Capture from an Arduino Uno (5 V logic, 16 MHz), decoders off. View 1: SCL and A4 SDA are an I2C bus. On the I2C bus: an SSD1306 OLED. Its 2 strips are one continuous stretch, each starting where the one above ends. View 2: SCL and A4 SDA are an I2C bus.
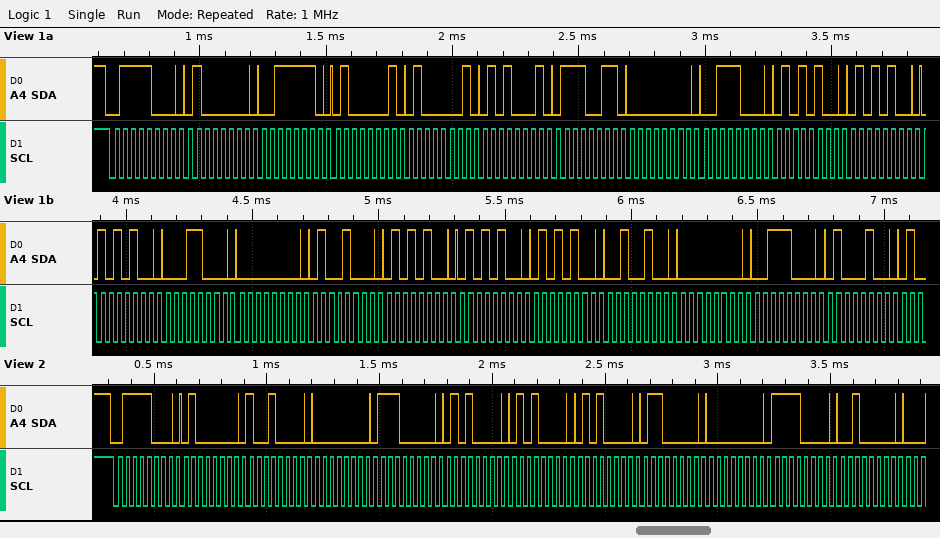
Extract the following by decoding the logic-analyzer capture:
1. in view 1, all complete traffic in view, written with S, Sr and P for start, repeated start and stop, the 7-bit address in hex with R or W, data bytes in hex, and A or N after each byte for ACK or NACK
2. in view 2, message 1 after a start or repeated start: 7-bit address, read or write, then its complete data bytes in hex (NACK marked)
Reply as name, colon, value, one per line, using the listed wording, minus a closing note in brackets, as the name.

in view 1, all complete traffic in view, written with S, Sr and P for start, repeated start and stop, the 7-bit address in hex with R or W, data bytes in hex, and A or N after each byte for ACK or NACK: S 3CW A 40 A 3E A 41 A 41 A 51 A 73 A 00 A 38 A 54 A 54 A 54 A 18 A 00 A 48 A 54 A 54 A 54 A 24 A 00 A 38 A 44 A
in view 2, message 1 after a start or repeated start: 7-bit address, read or write, then its complete data bytes in hex: 0x3C write: 40 90 00 E0 50 50 50 60 00 F0 20
